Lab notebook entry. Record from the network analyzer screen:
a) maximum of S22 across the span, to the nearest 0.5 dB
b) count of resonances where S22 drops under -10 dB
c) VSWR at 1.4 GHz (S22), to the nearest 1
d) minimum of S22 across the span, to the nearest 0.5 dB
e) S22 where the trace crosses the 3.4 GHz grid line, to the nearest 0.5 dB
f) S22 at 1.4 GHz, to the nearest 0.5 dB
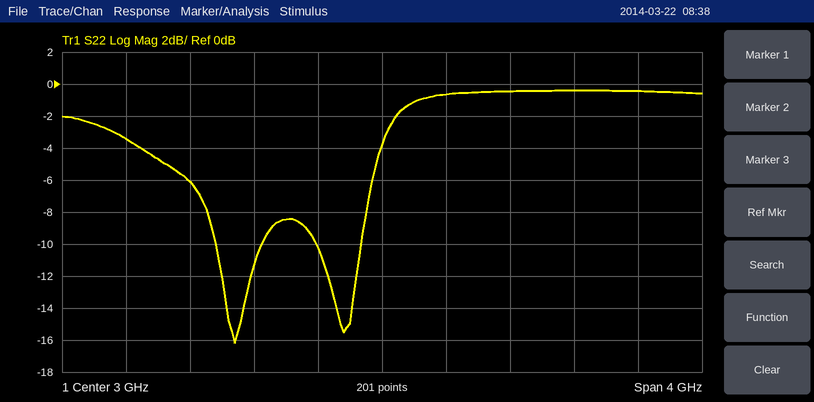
-0.5 dB
2
5
-16.0 dB
-0.5 dB
-3.5 dB
